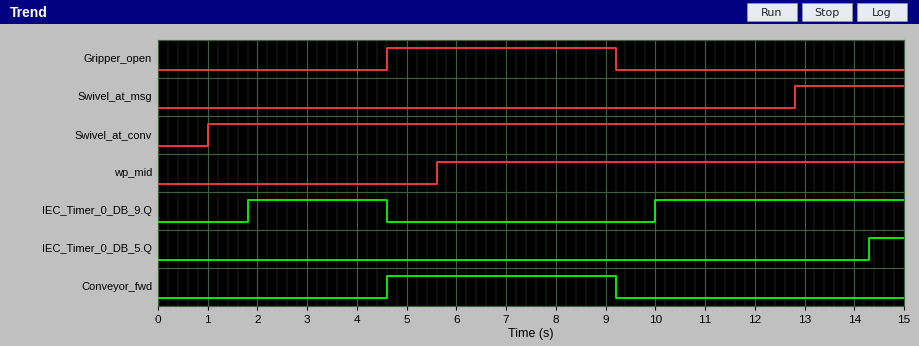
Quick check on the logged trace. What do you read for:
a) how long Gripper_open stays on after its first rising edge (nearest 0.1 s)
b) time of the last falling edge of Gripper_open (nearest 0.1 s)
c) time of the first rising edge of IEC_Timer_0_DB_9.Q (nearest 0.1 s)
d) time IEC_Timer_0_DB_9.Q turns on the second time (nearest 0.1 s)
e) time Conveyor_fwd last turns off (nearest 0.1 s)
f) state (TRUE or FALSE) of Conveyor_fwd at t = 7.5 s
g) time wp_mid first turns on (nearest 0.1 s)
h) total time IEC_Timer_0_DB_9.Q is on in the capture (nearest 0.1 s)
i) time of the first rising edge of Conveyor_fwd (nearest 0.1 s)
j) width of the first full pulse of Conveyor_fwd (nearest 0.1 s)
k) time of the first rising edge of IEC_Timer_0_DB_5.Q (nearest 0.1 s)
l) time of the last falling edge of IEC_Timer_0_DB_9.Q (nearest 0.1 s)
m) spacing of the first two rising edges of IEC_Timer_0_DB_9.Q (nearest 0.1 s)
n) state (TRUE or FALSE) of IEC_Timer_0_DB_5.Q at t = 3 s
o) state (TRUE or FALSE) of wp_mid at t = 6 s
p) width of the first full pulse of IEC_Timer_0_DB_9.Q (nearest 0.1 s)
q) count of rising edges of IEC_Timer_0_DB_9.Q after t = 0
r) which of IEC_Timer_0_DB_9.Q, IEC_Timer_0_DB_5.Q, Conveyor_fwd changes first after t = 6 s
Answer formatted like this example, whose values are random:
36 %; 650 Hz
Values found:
4.6 s; 9.2 s; 1.8 s; 10.0 s; 9.2 s; TRUE; 5.6 s; 7.8 s; 4.6 s; 4.6 s; 14.3 s; 4.6 s; 8.2 s; FALSE; TRUE; 2.8 s; 2; Conveyor_fwd
